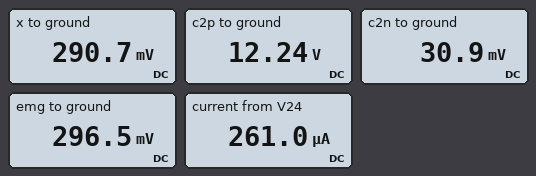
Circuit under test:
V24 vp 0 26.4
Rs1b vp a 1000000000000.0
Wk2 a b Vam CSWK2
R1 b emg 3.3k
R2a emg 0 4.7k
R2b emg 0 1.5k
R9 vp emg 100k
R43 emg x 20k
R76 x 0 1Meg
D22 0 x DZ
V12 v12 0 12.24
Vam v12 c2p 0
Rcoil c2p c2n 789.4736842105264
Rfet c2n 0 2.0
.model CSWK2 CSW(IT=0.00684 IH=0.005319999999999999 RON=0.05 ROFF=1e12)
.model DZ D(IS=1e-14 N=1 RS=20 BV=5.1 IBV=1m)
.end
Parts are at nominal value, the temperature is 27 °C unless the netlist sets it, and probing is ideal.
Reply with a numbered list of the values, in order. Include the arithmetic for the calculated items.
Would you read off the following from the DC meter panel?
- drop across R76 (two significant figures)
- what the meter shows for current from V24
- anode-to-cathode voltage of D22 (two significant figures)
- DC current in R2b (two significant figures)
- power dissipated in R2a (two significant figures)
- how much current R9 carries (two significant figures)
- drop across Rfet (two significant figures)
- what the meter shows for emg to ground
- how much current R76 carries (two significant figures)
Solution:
1. 290.7 mV = 290 mV
2. 261.0 µA
3. 0 V - 290.7 mV = -290 mV
4. (296.5 mV) / 1.5 kΩ = 200 µA
5. (296.5 mV)^2 / 4.7 kΩ = 19 µW
6. (26.4 V - 296.5 mV) / 100 kΩ = 260 µA
7. 30.9 mV = 31 mV
8. 296.5 mV
9. (290.7 mV) / 1 MΩ = 290 nA
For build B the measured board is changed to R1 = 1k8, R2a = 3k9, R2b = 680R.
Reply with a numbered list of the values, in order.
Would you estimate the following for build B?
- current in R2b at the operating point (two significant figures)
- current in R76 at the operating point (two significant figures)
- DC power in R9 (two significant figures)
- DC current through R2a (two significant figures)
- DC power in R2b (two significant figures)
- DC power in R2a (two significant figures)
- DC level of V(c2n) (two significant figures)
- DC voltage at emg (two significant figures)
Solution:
1. 220 µA
2. 150 nA
3. 6.9 mW
4. 39 µA
5. 34 µW
6. 5.9 µW
7. 31 mV
8. 150 mV
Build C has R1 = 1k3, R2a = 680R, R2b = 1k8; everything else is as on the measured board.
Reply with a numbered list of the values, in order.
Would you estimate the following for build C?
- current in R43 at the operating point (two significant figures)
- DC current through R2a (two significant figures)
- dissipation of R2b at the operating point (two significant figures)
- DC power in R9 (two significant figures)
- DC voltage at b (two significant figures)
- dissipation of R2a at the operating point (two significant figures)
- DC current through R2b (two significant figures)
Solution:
1. 130 nA
2. 190 µA
3. 9.3 µW
4. 6.9 mW
5. 130 mV
6. 25 µW
7. 72 µA
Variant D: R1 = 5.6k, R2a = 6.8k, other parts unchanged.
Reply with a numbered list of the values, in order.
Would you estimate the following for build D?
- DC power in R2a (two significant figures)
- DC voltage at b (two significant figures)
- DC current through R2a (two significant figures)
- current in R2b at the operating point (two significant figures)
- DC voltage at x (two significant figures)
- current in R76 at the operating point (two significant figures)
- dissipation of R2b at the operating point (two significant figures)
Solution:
1. 15 µW
2. 320 mV
3. 47 µA
4. 210 µA
5. 310 mV
6. 310 nA
7. 68 µW
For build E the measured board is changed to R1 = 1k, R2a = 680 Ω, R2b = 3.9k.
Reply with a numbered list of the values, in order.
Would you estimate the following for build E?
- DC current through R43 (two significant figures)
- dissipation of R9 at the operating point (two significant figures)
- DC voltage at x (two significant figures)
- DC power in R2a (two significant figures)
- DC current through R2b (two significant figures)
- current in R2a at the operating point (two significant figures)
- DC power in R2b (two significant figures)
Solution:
1. 150 nA
2. 6.9 mW
3. 150 mV
4. 34 µW
5. 39 µA
6. 220 µA
7. 5.9 µW
